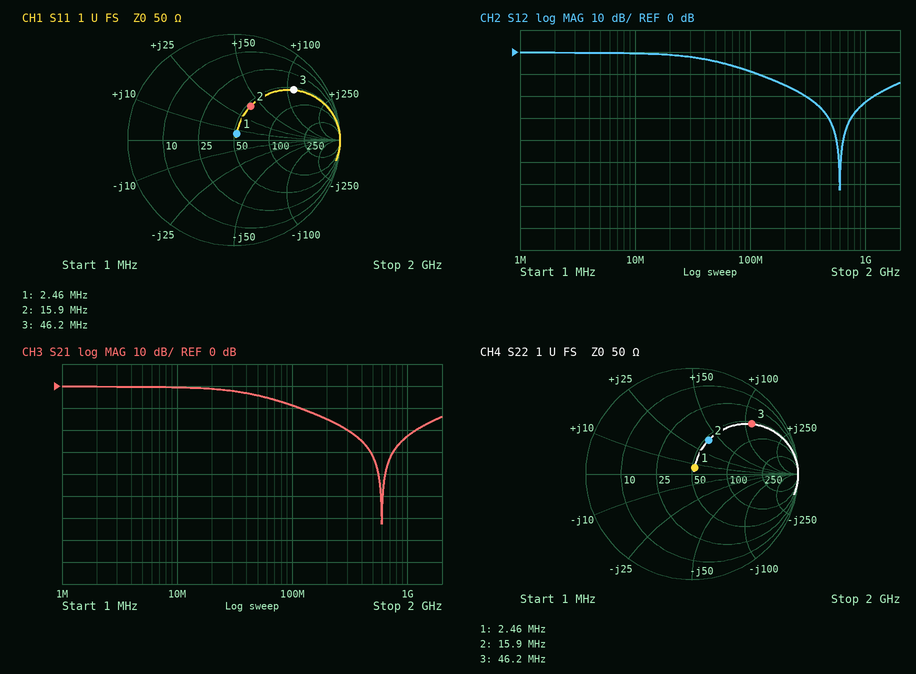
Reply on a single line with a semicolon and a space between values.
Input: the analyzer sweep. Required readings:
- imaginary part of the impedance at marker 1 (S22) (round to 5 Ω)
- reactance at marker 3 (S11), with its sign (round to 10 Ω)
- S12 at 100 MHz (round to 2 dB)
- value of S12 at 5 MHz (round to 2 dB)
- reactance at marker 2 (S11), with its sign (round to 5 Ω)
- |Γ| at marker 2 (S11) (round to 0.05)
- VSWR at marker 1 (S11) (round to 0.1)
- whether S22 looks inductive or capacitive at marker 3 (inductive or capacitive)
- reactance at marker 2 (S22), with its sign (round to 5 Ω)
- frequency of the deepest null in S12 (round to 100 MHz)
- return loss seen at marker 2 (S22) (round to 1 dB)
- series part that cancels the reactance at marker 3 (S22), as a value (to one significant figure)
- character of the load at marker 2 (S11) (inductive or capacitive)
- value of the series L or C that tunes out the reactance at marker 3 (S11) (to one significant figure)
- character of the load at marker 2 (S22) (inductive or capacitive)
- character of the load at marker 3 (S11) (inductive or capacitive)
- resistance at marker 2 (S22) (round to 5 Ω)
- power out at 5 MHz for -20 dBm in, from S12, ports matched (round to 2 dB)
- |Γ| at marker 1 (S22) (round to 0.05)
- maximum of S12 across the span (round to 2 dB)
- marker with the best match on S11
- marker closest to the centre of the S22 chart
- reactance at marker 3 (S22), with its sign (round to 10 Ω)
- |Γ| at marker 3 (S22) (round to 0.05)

+5 Ω; +110 Ω; -8 dB; 0 dB; +40 Ω; 0.35; 1.1; inductive; +40 Ω; 600 MHz; 9 dB; 30 pF; inductive; 30 pF; inductive; inductive; 55 Ω; -20 dBm; 0.05; 0 dB; marker 1; marker 1; +110 Ω; 0.75
